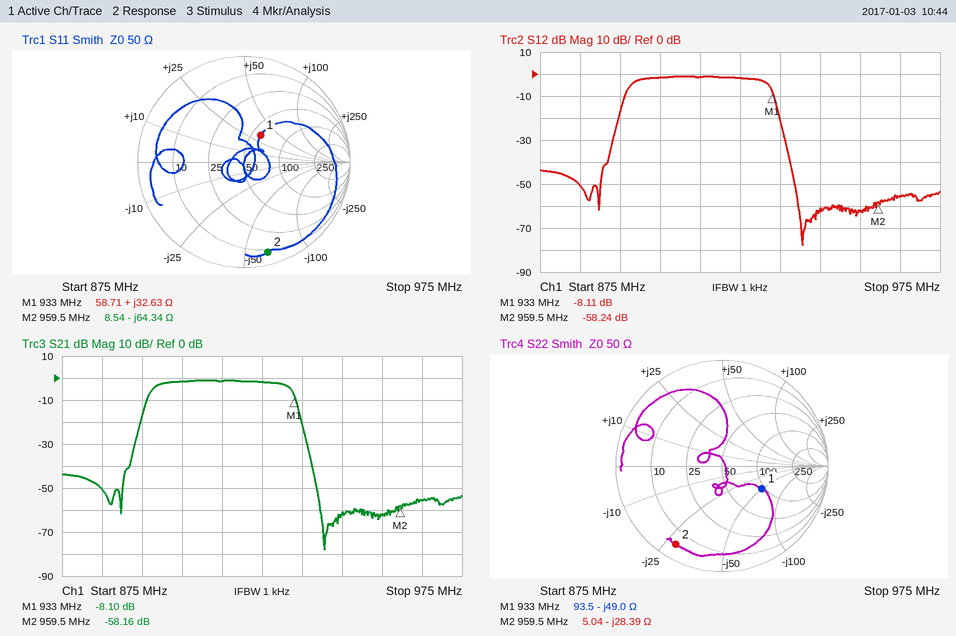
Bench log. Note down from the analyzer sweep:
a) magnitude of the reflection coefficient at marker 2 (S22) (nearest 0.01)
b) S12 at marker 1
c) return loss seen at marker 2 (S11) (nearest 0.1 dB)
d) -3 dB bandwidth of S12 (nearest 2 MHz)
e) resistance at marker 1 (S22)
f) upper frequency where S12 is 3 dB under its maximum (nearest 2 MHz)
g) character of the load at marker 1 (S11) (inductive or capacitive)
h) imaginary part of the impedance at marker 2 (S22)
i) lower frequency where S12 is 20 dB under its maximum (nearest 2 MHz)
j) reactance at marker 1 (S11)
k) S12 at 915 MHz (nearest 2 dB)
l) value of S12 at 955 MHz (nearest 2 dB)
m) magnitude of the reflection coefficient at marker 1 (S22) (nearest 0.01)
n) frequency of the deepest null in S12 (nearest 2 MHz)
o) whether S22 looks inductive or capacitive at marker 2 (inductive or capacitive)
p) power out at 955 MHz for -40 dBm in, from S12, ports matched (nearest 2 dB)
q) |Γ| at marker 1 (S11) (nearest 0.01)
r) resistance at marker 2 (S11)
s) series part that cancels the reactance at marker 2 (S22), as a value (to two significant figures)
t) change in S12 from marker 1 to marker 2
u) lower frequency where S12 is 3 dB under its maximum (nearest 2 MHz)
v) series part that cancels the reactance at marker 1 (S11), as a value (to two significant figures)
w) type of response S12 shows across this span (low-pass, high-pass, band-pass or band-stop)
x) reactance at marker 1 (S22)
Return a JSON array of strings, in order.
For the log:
["0.86", "-8.11 dB", "1.1 dB", "34 MHz", "93.5 Ω", "932 MHz", "inductive", "-28.39 Ω", "894 MHz", "+32.63 Ω", "-2 dB", "-62 dB", "0.43", "940 MHz", "capacitive", "-102 dBm", "0.30", "8.54 Ω", "4.7 nH", "-50.13 dB", "898 MHz", "5.2 pF", "band-pass", "-49.0 Ω"]
